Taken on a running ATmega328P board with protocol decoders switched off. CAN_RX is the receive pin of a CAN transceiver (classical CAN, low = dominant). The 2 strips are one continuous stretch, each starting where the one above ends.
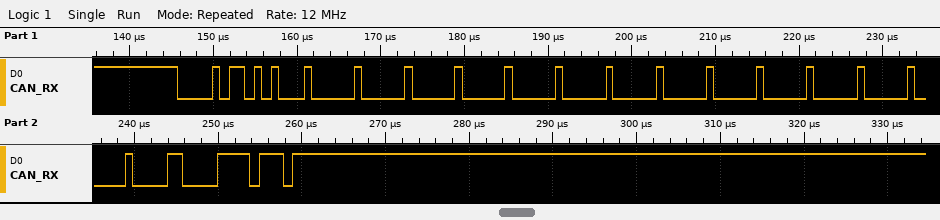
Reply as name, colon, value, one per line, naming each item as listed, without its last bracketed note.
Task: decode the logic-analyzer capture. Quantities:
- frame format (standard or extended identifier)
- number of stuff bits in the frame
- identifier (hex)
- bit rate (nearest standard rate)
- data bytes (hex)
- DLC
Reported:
frame format: standard
number of stuff bits in the frame: 13
identifier: 0x0B5
bit rate: 1000 kbit/s
data bytes: 00 00 00 00 00 00 00 00
DLC: 8
